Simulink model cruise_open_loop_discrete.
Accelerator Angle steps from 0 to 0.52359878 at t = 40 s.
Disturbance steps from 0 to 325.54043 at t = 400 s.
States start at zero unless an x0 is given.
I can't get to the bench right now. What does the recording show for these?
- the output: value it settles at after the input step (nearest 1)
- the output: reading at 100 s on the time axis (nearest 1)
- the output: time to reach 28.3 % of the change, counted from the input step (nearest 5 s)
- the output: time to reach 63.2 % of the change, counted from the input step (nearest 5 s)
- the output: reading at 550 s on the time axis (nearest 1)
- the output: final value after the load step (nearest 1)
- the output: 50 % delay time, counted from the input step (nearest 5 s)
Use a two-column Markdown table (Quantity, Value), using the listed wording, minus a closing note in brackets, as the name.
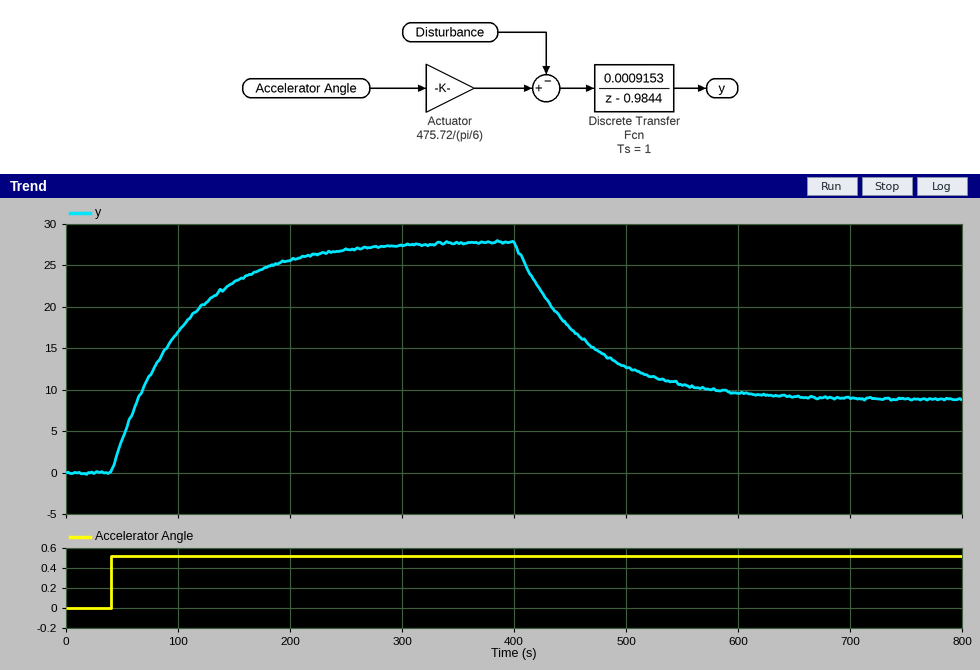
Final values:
| Quantity | Value |
|---|---|
| the output: value it settles at after the input step | 28 |
| the output: reading at 100 s on the time axis | 17 |
| the output: time to reach 28.3 % of the change, counted from the input step | 20 s |
| the output: time to reach 63.2 % of the change, counted from the input step | 65 s |
| the output: reading at 550 s on the time axis | 11 |
| the output: final value after the load step | 9 |
| the output: 50 % delay time, counted from the input step | 45 s |
